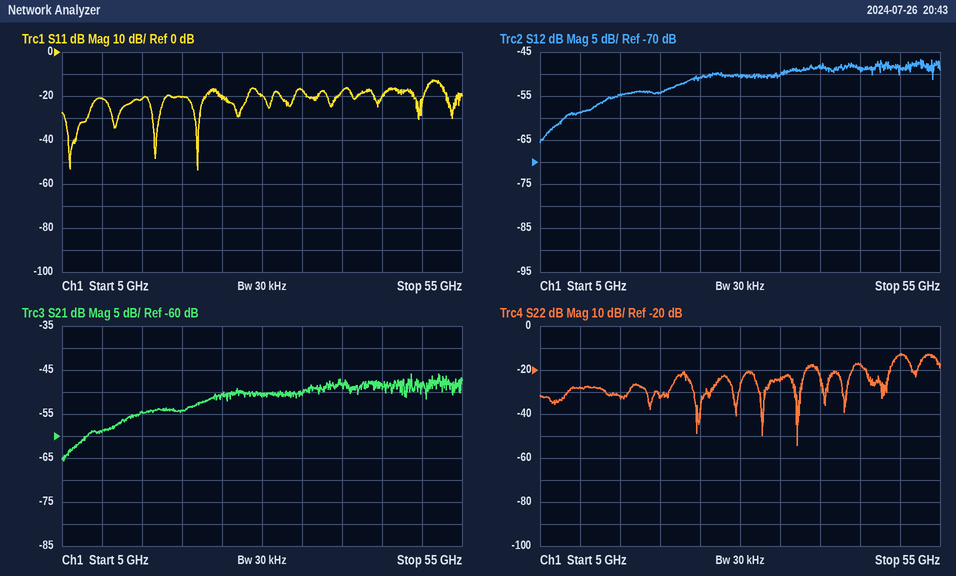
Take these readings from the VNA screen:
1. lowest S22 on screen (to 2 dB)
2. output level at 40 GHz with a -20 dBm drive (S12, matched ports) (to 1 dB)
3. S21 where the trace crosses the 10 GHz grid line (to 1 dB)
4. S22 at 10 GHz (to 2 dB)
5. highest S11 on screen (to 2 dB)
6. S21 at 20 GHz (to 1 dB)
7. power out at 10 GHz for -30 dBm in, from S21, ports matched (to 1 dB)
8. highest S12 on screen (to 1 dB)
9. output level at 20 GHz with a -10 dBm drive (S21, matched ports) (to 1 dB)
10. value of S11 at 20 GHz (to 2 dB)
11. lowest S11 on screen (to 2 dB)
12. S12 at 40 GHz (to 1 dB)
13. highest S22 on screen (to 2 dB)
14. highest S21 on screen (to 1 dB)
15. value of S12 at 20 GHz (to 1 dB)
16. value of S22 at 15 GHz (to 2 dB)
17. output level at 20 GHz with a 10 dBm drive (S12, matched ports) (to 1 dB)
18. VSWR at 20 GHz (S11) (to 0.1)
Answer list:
-54 dB
-68 dBm
-59 dB
-28 dB
-12 dB
-54 dB
-89 dBm
-47 dB
-64 dBm
-20 dB
-54 dB
-48 dB
-12 dB
-46 dB
-54 dB
-32 dB
-44 dBm
1.2
